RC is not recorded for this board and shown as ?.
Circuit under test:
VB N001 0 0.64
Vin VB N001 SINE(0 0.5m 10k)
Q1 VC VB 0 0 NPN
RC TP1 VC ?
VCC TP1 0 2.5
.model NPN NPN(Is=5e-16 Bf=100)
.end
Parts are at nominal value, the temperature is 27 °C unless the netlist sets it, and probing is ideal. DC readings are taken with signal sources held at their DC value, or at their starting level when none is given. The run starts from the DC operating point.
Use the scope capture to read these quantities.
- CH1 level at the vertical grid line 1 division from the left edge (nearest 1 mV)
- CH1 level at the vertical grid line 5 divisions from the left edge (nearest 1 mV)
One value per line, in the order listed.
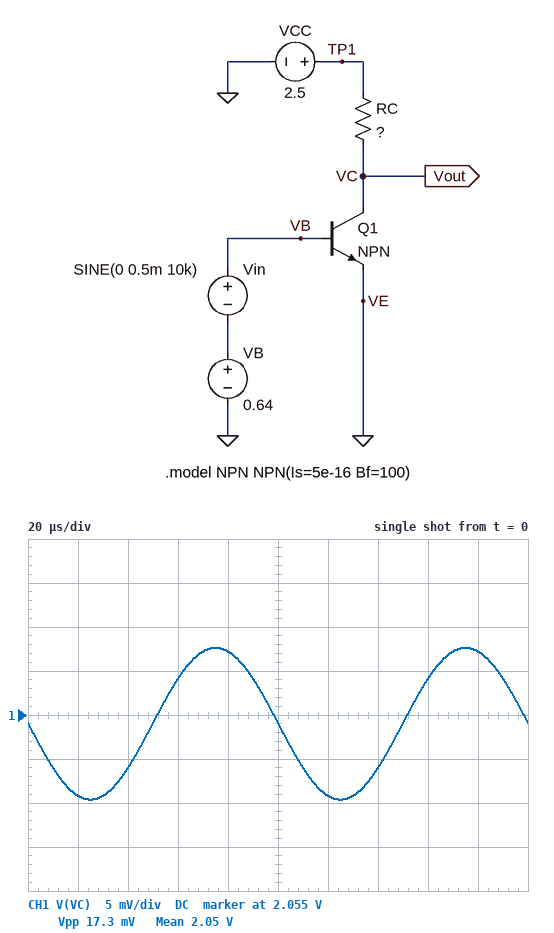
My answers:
2.046 V
2.054 V
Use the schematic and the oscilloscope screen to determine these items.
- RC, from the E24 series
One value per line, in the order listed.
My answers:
16 kΩ
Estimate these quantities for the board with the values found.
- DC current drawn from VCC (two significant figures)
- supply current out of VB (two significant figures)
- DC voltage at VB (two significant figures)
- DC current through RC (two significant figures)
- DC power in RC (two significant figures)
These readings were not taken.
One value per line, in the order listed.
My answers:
28 µA
280 nA
640 mV
28 µA
12 µW
